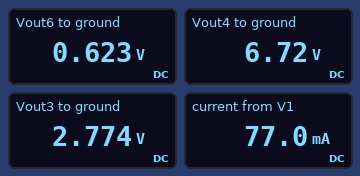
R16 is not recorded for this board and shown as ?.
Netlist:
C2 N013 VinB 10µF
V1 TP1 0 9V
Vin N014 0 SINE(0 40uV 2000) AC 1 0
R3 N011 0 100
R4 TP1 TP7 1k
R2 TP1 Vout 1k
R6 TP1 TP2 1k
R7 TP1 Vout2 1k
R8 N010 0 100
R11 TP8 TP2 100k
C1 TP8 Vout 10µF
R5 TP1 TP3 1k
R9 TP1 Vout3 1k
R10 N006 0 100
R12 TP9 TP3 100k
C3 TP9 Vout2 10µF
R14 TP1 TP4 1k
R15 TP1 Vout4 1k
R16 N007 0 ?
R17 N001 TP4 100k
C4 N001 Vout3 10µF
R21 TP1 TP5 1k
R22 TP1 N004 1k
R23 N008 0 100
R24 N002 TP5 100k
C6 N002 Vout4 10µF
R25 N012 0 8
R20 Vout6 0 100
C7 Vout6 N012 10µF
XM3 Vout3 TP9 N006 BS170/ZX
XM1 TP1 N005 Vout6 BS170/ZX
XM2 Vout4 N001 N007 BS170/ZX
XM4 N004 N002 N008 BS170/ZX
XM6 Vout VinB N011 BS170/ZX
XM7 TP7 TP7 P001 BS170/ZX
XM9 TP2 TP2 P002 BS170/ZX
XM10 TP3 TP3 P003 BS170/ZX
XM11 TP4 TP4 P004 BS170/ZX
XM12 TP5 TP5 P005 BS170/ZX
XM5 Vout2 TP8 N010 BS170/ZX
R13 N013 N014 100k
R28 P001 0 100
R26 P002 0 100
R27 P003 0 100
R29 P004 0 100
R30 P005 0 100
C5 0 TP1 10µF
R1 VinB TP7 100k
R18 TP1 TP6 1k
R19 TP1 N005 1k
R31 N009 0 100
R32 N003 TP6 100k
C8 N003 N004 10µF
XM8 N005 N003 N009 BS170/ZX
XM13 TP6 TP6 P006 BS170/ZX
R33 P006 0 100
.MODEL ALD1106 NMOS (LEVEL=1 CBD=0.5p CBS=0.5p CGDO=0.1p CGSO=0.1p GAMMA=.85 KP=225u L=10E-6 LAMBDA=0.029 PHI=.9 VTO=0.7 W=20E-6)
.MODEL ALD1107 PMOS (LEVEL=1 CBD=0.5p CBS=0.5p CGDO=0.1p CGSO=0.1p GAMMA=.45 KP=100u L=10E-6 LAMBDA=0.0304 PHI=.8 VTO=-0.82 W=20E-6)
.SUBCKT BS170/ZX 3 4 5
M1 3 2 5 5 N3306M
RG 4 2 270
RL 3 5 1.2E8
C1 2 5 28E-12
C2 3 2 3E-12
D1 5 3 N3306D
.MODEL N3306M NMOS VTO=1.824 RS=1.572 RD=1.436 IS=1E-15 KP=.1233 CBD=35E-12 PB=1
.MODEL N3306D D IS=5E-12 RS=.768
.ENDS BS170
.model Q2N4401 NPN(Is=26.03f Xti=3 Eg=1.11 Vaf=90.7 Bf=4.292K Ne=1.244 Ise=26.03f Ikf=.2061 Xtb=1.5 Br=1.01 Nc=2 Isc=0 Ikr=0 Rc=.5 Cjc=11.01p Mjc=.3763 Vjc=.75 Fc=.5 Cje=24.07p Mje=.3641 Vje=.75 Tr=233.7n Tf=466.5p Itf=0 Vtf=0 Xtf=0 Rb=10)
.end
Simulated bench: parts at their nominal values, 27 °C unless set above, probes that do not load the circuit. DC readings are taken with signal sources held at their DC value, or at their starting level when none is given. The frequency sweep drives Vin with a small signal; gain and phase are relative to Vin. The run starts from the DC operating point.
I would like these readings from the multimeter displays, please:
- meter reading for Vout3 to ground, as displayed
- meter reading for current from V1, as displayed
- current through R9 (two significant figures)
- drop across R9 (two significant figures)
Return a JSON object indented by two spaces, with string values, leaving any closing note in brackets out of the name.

{
  "meter reading for Vout3 to ground, as displayed": "2.774 V",
  "meter reading for current from V1, as displayed": "77.0 mA",
  "current through R9": "6.2 mA",
  "drop across R9": "6.2 V"
}
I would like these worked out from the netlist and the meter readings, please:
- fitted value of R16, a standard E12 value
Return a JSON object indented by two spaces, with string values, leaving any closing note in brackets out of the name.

{
  "fitted value of R16, a standard E12 value": "330 Ω"
}
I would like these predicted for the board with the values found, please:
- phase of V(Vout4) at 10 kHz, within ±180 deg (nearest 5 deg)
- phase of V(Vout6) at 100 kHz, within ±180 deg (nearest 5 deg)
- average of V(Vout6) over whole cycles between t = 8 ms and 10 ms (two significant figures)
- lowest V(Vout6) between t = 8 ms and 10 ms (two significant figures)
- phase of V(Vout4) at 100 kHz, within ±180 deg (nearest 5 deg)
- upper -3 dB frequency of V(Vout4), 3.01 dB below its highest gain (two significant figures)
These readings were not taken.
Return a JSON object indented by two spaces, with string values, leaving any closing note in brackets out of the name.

{
  "phase of V(Vout4) at 10 kHz, within ±180 deg": "-5 deg",
  "phase of V(Vout6) at 100 kHz, within ±180 deg": "-55 deg",
  "average of V(Vout6) over whole cycles between t = 8 ms and 10 ms": "1.2 V",
  "lowest V(Vout6) between t = 8 ms and 10 ms": "990 mV",
  "phase of V(Vout4) at 100 kHz, within ±180 deg": "-50 deg",
  "upper -3 dB frequency of V(Vout4), 3.01 dB below its highest gain": "96 kHz"
}
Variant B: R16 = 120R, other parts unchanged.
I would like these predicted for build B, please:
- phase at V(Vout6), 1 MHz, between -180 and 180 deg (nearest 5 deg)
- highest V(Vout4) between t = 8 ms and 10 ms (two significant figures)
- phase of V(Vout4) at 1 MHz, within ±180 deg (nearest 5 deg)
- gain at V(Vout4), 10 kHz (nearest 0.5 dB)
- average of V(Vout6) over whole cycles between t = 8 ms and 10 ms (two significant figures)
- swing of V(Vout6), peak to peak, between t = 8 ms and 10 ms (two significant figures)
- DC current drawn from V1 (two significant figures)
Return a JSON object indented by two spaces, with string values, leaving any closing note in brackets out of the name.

{
  "phase at V(Vout6), 1 MHz, between -180 and 180 deg": "-170 deg",
  "highest V(Vout4) between t = 8 ms and 10 ms": "3.7 V",
  "phase of V(Vout4) at 1 MHz, within ±180 deg": "-135 deg",
  "gain at V(Vout4), 10 kHz": "64.0 dB",
  "average of V(Vout6) over whole cycles between t = 8 ms and 10 ms": "2.5 V",
  "swing of V(Vout6), peak to peak, between t = 8 ms and 10 ms": "1.2 V",
  "DC current drawn from V1": "80 mA"
}
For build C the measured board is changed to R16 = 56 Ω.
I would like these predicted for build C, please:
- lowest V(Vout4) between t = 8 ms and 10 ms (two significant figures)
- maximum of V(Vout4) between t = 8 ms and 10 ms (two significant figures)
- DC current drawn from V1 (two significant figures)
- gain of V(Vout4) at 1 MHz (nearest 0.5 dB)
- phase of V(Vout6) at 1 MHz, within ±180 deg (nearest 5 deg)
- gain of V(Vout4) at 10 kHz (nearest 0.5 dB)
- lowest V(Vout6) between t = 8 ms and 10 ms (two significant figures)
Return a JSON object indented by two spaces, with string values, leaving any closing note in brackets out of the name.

{
  "lowest V(Vout4) between t = 8 ms and 10 ms": "660 mV",
  "maximum of V(Vout4) between t = 8 ms and 10 ms": "670 mV",
  "DC current drawn from V1": "83 mA",
  "gain of V(Vout4) at 1 MHz": "20.5 dB",
  "phase of V(Vout6) at 1 MHz, within ±180 deg": "-160 deg",
  "gain of V(Vout4) at 10 kHz": "42.0 dB",
  "lowest V(Vout6) between t = 8 ms and 10 ms": "580 mV"
}
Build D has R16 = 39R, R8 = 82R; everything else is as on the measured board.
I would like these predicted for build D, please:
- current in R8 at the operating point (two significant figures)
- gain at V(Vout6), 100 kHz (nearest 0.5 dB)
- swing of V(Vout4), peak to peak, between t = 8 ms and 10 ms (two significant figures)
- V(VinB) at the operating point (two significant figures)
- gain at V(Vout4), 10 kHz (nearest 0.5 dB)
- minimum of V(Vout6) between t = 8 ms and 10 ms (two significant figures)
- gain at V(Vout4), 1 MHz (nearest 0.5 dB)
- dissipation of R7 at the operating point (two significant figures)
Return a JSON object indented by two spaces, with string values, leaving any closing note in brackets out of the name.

{
  "current in R8 at the operating point": "7.3 mA",
  "gain at V(Vout6), 100 kHz": "56.0 dB",
  "swing of V(Vout4), peak to peak, between t = 8 ms and 10 ms": "5.6 mV",
  "V(VinB) at the operating point": "2.8 V",
  "gain at V(Vout4), 10 kHz": "37.0 dB",
  "minimum of V(Vout6) between t = 8 ms and 10 ms": "590 mV",
  "gain at V(Vout4), 1 MHz": "15.5 dB",
  "dissipation of R7 at the operating point": "53 mW"
}
